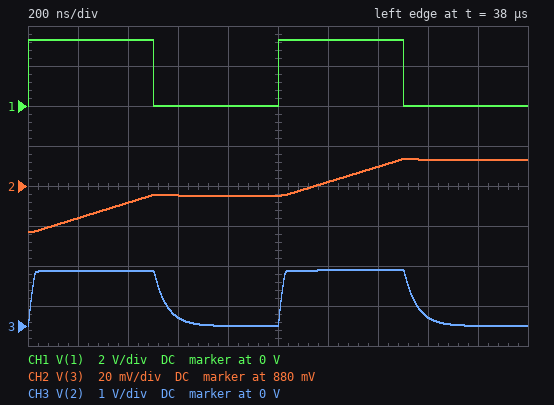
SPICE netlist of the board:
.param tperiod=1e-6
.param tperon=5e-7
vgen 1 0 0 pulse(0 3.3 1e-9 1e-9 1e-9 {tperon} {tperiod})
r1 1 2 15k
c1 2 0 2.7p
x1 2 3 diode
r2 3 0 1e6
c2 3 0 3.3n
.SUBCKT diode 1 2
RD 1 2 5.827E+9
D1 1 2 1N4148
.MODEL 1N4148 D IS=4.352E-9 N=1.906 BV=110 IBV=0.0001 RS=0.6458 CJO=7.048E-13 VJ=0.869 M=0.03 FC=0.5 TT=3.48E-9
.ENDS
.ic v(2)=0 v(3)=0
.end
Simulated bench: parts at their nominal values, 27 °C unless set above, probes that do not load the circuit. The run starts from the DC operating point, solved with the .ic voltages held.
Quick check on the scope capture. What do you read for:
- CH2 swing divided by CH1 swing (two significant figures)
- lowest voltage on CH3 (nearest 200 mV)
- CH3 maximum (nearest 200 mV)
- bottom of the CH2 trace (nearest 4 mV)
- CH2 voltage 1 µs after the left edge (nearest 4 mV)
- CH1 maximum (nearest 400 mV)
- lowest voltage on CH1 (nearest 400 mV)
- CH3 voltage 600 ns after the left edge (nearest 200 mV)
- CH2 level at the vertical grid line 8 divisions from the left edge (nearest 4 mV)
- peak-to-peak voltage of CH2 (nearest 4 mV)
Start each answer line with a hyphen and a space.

- 0.011
- 0 V
- 1.4 V
- 856 mV
- 876 mV
- 3.2 V
- 0 V
- 200 mV
- 892 mV
- 36 mV
